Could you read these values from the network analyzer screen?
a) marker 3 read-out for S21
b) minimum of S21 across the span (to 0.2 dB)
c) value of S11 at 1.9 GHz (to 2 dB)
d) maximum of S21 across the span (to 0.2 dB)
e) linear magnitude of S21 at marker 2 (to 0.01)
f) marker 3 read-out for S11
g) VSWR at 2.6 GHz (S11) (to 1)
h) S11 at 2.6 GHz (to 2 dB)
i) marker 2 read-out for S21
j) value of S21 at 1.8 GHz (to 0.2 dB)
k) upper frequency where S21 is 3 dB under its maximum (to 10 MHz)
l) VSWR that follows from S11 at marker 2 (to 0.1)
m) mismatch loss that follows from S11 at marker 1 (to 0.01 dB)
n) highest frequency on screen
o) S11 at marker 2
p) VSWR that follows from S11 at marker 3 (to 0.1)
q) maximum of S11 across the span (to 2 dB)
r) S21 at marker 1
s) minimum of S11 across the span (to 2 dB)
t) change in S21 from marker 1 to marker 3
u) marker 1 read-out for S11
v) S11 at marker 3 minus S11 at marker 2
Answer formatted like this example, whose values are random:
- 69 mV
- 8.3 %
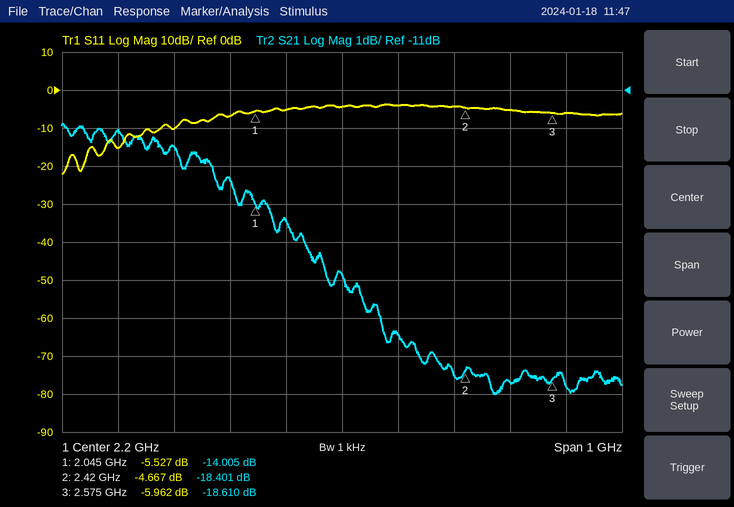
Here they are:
- -18.610 dB
- -19.0 dB
- -10 dB
- -11.8 dB
- 0.12
- -5.962 dB
- 3
- -6 dB
- -18.401 dB
- -12.0 dB
- 2.11 GHz
- 3.8
- 1.43 dB
- 2.7 GHz
- -4.667 dB
- 3.0
- -4 dB
- -14.005 dB
- -22 dB
- -4.605 dB
- -5.527 dB
- -1.295 dB
